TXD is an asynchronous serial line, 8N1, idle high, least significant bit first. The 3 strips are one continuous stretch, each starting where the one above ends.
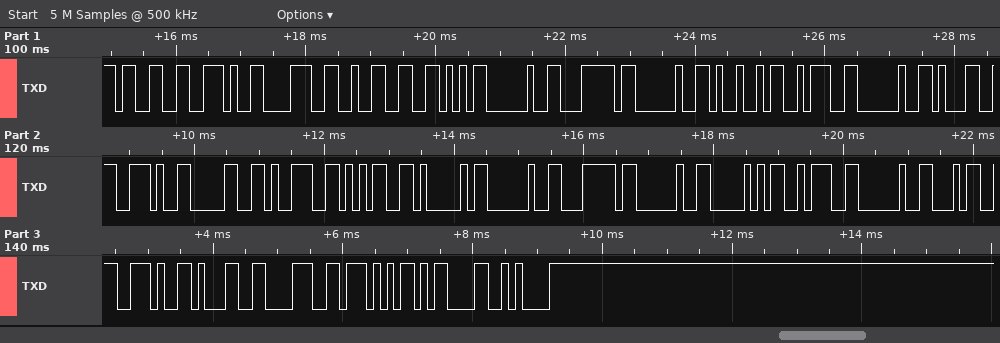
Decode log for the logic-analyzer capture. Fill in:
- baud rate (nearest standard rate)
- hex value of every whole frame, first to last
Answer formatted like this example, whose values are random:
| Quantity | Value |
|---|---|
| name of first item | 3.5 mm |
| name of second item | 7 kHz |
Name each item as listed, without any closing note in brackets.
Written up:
| Quantity | Value |
|---|---|
| baud rate | 9600 baud |
| hex value of every whole frame, first to last | 33 2E 38 32 56 20 7C 20 49 3A 20 31 2E 30 39 35 41 20 7C 20 50 3A 20 34 2E 31 38 57 0D 0A |
